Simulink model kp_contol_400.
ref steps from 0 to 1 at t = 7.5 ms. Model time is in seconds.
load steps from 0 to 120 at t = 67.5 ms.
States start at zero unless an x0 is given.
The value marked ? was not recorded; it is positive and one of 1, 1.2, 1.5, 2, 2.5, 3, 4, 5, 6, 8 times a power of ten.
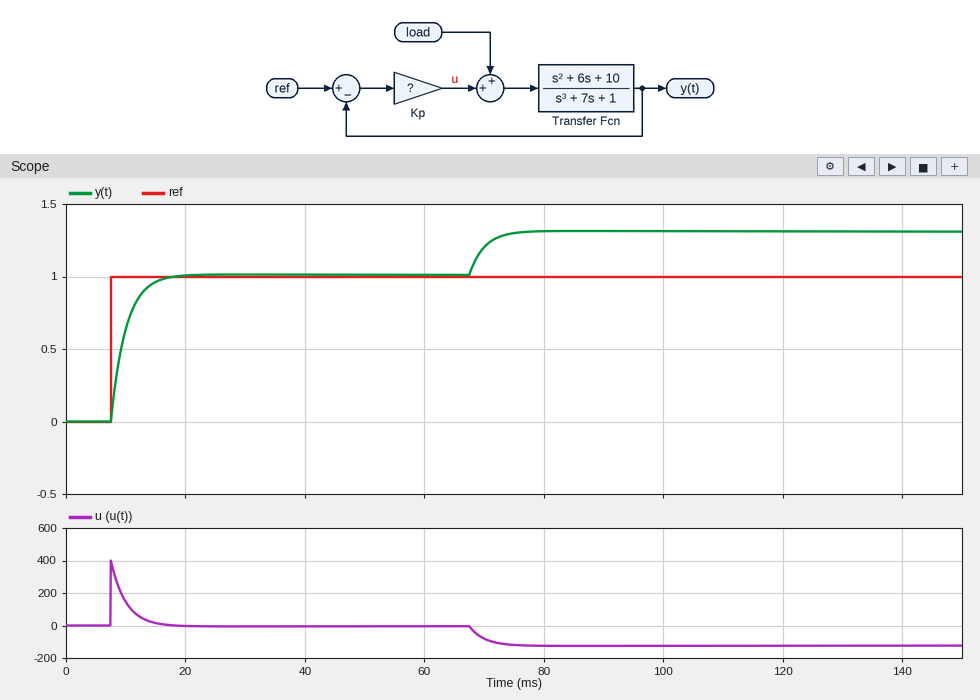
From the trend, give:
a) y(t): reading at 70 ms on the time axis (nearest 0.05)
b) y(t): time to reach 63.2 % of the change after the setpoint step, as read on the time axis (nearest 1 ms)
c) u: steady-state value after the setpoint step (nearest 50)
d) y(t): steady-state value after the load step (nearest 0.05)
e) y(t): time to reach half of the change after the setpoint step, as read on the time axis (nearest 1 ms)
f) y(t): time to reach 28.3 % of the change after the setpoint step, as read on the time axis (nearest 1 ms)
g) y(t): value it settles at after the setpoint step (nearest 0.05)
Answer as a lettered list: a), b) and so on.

a) 1.20
b) 10 ms
c) 0
d) 1.30
e) 9 ms
f) 8 ms
g) 1.00
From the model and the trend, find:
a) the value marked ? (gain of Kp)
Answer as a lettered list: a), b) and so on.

a) 400
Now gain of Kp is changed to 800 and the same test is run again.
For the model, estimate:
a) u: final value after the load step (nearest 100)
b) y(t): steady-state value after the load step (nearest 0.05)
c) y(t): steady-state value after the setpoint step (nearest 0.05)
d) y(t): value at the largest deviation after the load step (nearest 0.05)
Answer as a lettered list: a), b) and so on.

a) -100
b) 1.15
c) 1.00
d) 1.15
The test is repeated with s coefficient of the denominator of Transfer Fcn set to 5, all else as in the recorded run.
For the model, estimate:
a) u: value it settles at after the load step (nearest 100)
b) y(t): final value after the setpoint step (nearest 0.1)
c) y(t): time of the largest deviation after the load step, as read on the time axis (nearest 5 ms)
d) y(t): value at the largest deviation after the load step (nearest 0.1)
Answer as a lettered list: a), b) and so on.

a) -100
b) 1.0
c) 85 ms
d) 1.3
